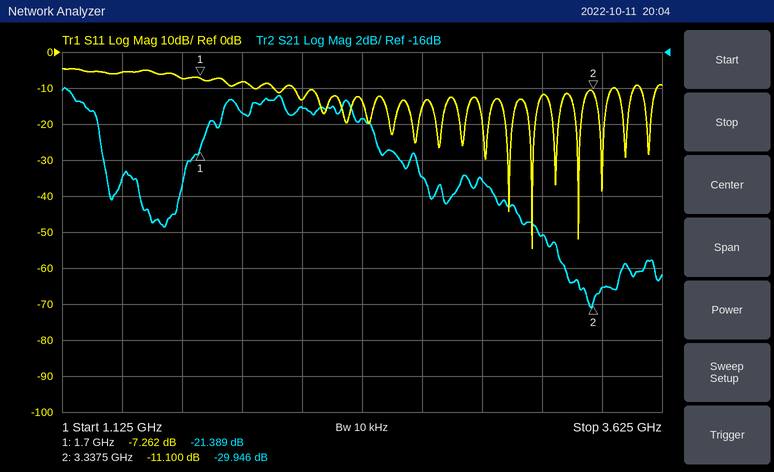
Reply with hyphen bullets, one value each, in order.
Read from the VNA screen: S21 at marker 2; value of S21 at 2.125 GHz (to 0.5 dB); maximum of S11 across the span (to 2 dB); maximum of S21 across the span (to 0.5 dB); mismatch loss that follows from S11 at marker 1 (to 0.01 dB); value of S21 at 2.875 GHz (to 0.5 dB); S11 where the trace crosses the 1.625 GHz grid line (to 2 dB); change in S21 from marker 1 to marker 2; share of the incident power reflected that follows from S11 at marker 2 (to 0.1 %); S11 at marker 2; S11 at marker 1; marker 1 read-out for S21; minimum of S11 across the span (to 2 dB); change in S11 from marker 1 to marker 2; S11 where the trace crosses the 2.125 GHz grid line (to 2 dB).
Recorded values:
- -29.946 dB
- -19.0 dB
- -4 dB
- -18.0 dB
- 0.90 dB
- -23.0 dB
- -8 dB
- -8.557 dB
- 7.8 %
- -11.100 dB
- -7.262 dB
- -21.389 dB
- -54 dB
- -3.838 dB
- -14 dB
